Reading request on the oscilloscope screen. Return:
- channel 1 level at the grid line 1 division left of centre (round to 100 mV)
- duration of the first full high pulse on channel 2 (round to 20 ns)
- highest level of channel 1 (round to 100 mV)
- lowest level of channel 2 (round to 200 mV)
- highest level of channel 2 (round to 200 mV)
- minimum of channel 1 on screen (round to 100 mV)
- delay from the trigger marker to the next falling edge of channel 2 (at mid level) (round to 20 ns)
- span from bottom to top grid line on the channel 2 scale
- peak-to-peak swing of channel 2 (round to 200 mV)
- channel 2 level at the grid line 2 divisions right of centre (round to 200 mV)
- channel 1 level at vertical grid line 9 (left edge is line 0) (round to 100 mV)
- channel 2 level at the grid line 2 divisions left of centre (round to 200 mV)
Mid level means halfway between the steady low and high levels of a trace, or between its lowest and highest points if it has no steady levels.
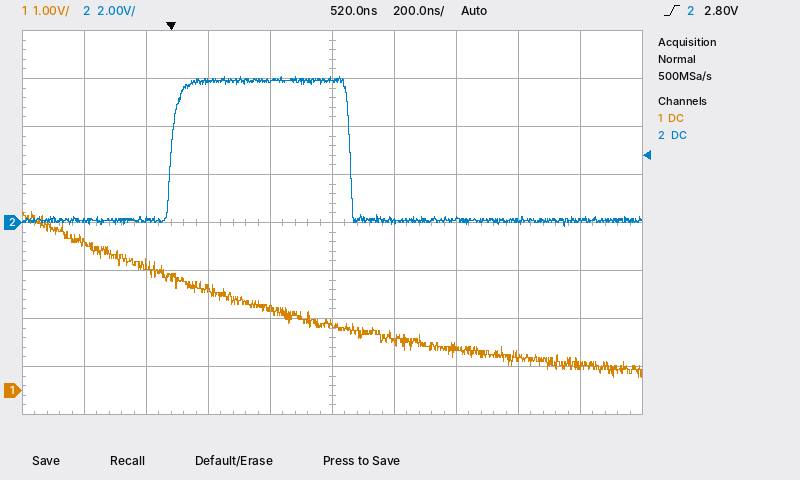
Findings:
1.7 V
580 ns
3.7 V
-200 mV
6.0 V
300 mV
580 ns
16 V
6.2 V
200 mV
500 mV
5.8 V
